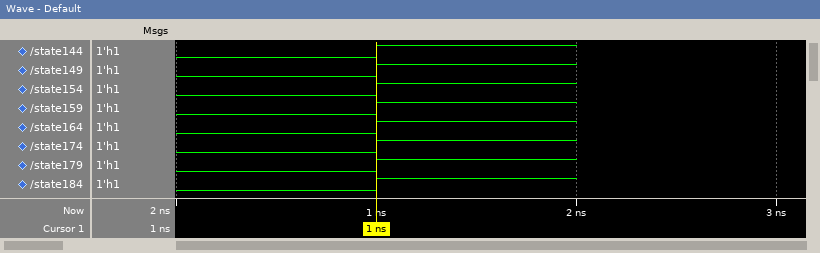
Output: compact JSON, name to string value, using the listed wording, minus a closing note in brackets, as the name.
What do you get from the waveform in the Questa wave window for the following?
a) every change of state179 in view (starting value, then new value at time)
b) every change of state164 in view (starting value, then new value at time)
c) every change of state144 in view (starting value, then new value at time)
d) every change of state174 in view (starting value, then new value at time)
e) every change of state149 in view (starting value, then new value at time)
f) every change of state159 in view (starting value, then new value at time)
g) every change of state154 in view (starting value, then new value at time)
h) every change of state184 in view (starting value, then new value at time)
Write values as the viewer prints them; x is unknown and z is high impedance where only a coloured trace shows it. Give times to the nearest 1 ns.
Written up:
{"every change of state179 in view": "0, 1 at 1 ns", "every change of state164 in view": "0, 1 at 1 ns", "every change of state144 in view": "0, 1 at 1 ns", "every change of state174 in view": "0, 1 at 1 ns", "every change of state149 in view": "0, 1 at 1 ns", "every change of state159 in view": "0, 1 at 1 ns", "every change of state154 in view": "0, 1 at 1 ns", "every change of state184 in view": "0, 1 at 1 ns"}
